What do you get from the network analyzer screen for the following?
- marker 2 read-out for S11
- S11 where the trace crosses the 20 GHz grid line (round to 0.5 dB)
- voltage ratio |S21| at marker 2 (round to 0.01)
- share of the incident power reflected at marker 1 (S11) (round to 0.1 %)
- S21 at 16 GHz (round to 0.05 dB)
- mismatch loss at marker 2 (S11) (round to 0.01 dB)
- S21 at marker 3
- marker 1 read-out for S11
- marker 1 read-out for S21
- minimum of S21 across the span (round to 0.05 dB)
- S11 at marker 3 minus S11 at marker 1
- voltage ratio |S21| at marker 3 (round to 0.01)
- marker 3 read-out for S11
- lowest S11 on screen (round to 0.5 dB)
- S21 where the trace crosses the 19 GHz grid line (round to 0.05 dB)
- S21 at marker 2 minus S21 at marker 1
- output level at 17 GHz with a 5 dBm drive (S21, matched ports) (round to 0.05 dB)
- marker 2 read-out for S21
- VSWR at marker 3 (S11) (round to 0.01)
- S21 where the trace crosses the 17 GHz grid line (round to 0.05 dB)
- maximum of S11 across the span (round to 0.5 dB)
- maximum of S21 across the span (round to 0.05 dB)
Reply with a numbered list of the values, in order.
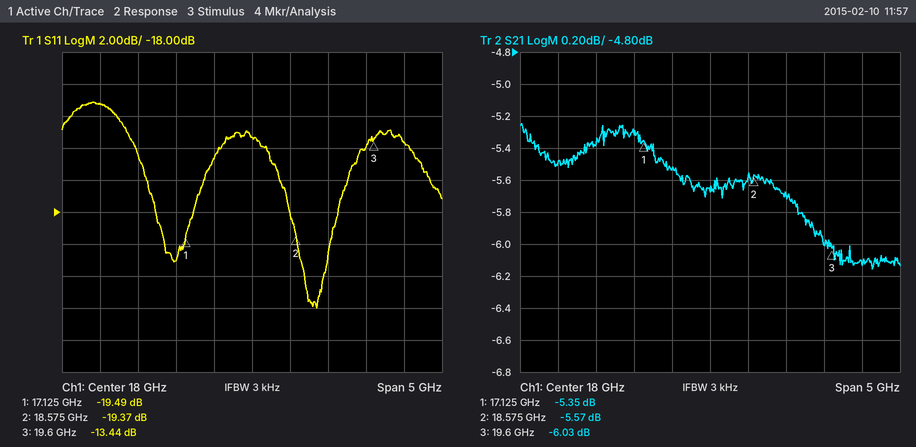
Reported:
1. -19.37 dB
2. -13.5 dB
3. 0.53
4. 1.1 %
5. -5.50 dB
6. 0.05 dB
7. -6.03 dB
8. -19.49 dB
9. -5.35 dB
10. -6.15 dB
11. 6.05 dB
12. 0.50
13. -13.44 dB
14. -24.0 dB
15. -5.70 dB
16. -0.22 dB
17. -0.30 dBm
18. -5.57 dB
19. 1.54
20. -5.30 dB
21. -11.0 dB
22. -5.25 dB
